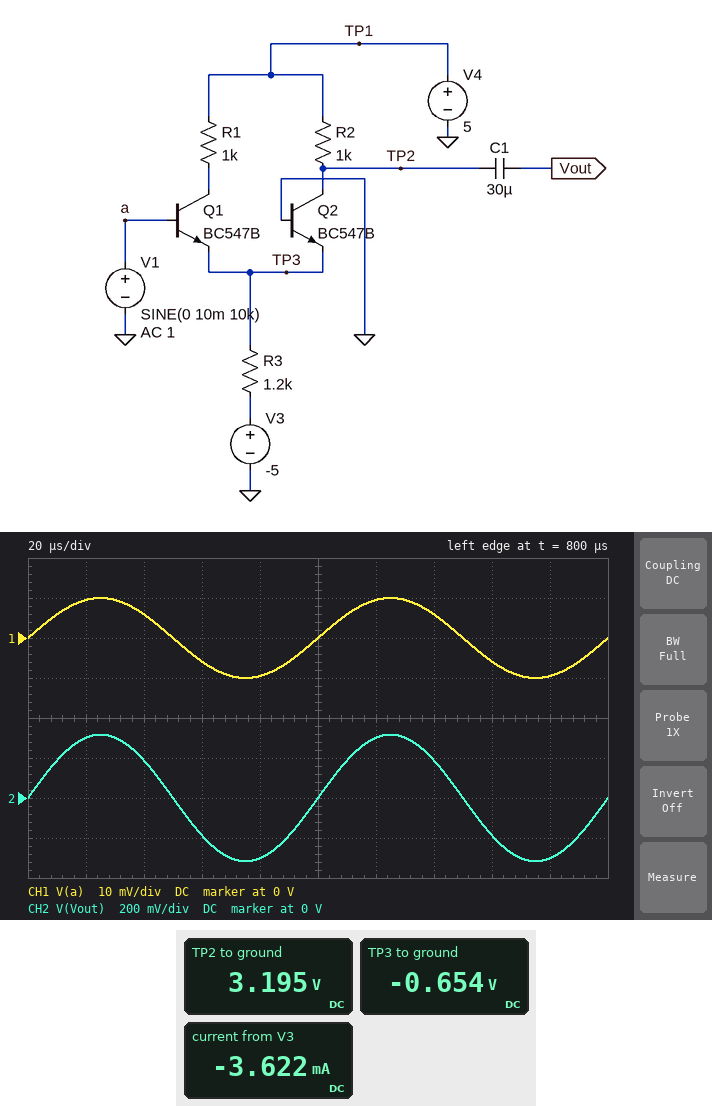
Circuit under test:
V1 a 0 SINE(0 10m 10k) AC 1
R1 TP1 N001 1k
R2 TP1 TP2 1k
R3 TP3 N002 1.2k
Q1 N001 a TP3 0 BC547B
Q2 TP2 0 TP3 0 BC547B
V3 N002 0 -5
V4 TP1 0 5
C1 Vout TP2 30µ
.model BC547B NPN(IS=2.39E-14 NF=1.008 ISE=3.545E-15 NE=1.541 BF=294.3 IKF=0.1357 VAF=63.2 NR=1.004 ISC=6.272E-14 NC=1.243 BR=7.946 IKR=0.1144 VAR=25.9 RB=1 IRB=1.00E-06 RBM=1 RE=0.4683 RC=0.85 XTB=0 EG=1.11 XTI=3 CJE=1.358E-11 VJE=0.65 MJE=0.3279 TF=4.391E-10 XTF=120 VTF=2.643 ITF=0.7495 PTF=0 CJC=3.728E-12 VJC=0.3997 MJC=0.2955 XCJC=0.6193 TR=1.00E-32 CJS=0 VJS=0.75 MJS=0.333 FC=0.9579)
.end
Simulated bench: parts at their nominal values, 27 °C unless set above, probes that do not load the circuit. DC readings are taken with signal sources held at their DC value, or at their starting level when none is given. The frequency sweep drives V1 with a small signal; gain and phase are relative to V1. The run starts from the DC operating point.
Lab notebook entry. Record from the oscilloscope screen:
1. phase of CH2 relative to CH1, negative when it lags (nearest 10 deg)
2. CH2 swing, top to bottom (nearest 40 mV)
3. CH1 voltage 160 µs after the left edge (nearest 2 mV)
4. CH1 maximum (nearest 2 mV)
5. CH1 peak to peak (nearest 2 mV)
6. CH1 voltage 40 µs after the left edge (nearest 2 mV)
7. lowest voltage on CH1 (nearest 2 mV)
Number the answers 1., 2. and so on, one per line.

1. 0 deg
2. 640 mV
3. -6 mV
4. 10 mV
5. 20 mV
6. 6 mV
7. -10 mV
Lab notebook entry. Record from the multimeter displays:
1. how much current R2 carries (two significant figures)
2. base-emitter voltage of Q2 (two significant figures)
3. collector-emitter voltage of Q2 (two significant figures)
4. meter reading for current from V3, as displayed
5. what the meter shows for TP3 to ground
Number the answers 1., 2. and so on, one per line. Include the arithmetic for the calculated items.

1. (5 V - 3.195 V) / 1 kΩ = 1.8 mA
2. 0 V - (-654 mV) = 650 mV
3. 3.195 V - (-654 mV) = 3.8 V
4. -3.622 mA
5. -0.654 V
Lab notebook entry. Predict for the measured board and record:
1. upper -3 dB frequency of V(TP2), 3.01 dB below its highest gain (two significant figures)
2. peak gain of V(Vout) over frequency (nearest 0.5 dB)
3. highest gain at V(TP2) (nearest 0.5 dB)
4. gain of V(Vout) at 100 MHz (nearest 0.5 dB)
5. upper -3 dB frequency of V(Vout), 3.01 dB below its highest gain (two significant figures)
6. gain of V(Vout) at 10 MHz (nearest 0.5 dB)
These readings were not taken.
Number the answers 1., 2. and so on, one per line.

1. 80 MHz
2. 30.0 dB
3. 30.0 dB
4. 26.0 dB
5. 80 MHz
6. 30.0 dB
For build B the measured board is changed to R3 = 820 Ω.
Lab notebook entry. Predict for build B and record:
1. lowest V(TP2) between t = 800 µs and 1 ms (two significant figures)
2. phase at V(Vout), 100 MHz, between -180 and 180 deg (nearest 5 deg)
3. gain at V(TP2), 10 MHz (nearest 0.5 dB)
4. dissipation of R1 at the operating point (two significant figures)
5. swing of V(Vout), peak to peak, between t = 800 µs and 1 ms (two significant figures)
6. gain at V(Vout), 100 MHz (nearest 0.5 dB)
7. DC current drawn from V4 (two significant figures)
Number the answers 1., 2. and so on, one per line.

1. 1.9 V
2. -60 deg
3. 33.0 dB
4. 6.9 mW
5. 900 mV
6. 28.5 dB
7. 5.3 mA
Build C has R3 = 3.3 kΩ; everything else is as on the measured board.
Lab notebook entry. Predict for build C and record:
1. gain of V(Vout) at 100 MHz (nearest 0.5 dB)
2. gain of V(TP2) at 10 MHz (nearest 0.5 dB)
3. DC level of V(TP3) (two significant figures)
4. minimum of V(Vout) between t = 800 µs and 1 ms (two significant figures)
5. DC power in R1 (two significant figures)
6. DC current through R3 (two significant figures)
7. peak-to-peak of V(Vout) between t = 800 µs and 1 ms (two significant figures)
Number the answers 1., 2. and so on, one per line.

1. 18.0 dB
2. 21.5 dB
3. -630 mV
4. -120 mV
5. 440 µW
6. 1.3 mA
7. 240 mV
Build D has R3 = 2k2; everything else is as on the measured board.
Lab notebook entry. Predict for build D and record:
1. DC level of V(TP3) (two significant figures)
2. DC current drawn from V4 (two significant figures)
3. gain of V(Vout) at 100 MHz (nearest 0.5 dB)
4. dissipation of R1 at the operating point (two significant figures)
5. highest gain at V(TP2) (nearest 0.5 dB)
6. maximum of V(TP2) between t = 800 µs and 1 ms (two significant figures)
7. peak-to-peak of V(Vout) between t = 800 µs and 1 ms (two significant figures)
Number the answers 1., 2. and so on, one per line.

1. -640 mV
2. 2.0 mA
3. 21.5 dB
4. 980 µW
5. 25.0 dB
6. 4.2 V
7. 360 mV
